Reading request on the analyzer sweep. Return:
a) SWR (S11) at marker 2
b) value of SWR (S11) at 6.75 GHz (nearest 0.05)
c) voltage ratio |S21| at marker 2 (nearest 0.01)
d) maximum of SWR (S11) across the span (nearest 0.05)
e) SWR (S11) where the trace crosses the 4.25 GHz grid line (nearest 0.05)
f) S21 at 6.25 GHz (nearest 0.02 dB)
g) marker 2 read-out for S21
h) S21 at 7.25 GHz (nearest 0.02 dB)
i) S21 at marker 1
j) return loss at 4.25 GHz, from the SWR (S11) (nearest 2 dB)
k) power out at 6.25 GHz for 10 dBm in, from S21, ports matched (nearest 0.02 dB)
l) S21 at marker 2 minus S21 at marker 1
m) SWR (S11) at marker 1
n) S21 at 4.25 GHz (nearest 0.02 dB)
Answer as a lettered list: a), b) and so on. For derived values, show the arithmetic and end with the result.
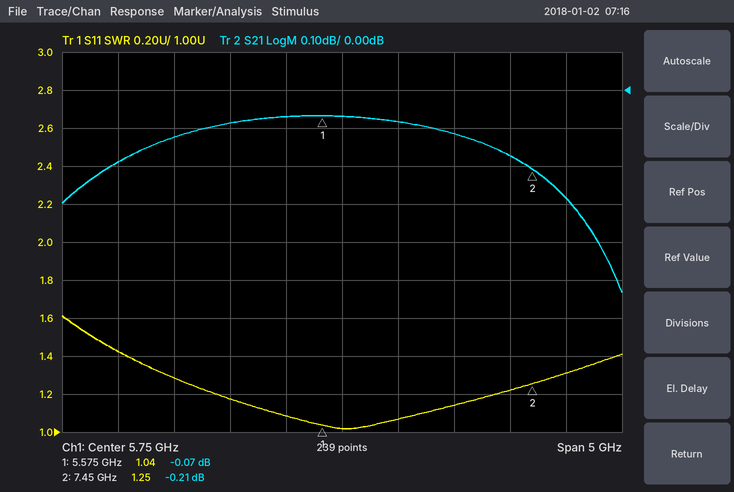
a) 1.25
b) 1.15
c) 10^(-0.21/20) ≈ 0.98
d) 1.60
e) 1.30
f) -0.08 dB
g) -0.21 dB
h) -0.18 dB
i) -0.07 dB
j) −20 log10((1.3 − 1)/(1.3 + 1)) ≈ 18 dB
k) 10 dBm + (-0.08 dB) = 9.92 dBm
l) -0.21 − (-0.07) = -0.14 dB
m) 1.04
n) -0.12 dB
